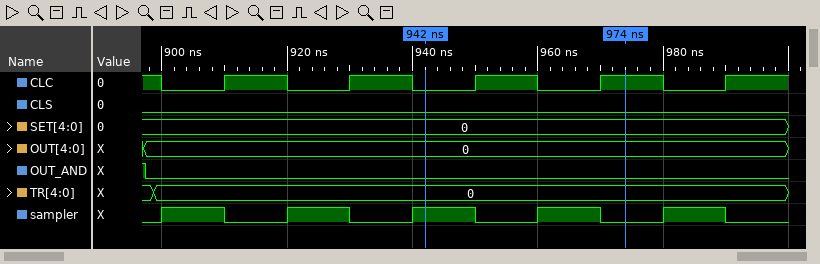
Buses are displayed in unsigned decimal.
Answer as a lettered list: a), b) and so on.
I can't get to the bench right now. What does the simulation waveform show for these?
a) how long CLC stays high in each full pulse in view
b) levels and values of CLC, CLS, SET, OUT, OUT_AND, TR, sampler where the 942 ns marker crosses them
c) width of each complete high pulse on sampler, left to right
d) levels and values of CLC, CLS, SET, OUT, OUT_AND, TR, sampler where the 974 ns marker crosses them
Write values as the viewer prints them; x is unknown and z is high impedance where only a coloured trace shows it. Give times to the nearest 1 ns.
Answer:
a) 10 ns, 10 ns, 10 ns, 10 ns
b) CLC=0, CLS=0, SET=0, OUT=0, OUT_AND=0, TR=0, sampler=1
c) 10 ns, 10 ns, 10 ns, 10 ns, 10 ns
d) CLC=1, CLS=0, SET=0, OUT=0, OUT_AND=0, TR=0, sampler=0
